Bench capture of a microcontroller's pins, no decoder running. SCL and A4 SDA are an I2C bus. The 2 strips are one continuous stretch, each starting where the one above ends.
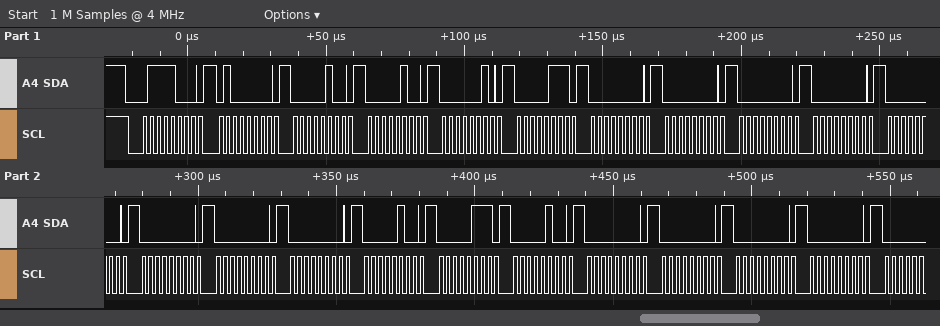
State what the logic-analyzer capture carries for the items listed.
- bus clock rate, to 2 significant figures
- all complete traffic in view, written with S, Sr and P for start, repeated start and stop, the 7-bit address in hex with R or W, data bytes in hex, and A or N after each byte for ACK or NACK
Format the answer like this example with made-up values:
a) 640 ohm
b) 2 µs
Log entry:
a) 400 kHz
b) S 3CW A 40 A 04 A 04 A 02 A 07 A 00 A 00 A 00 A 00 A 00 A 00 A 00 A 00 A 04 A 07 A 04 A 00 A 00 A 00 A 00 A
